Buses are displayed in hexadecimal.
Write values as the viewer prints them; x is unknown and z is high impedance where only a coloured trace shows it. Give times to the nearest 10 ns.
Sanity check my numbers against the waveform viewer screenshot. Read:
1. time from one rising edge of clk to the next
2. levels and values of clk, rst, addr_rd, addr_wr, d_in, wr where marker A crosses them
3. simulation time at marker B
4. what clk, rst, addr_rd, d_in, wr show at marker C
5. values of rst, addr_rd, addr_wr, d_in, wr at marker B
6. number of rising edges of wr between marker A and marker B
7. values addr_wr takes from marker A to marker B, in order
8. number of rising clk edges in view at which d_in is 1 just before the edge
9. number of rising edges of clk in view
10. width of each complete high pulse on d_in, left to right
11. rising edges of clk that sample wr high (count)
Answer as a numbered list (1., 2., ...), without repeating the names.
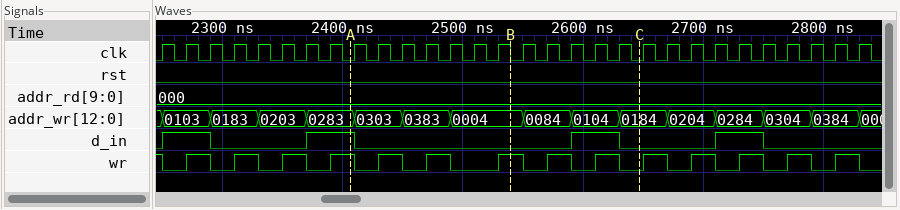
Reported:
1. 20 ns
2. clk=0, rst=0, addr_rd=000, addr_wr=0283, d_in=1, wr=1
3. 2540 ns
4. clk=0, rst=0, addr_rd=000, d_in=0, wr=0
5. rst=0, addr_rd=000, addr_wr=0004, d_in=0, wr=1
6. 3
7. 0283, 0303, 0383, 0004
8. 8
9. 30
10. 40 ns, 40 ns, 40 ns, 40 ns
11. 15
